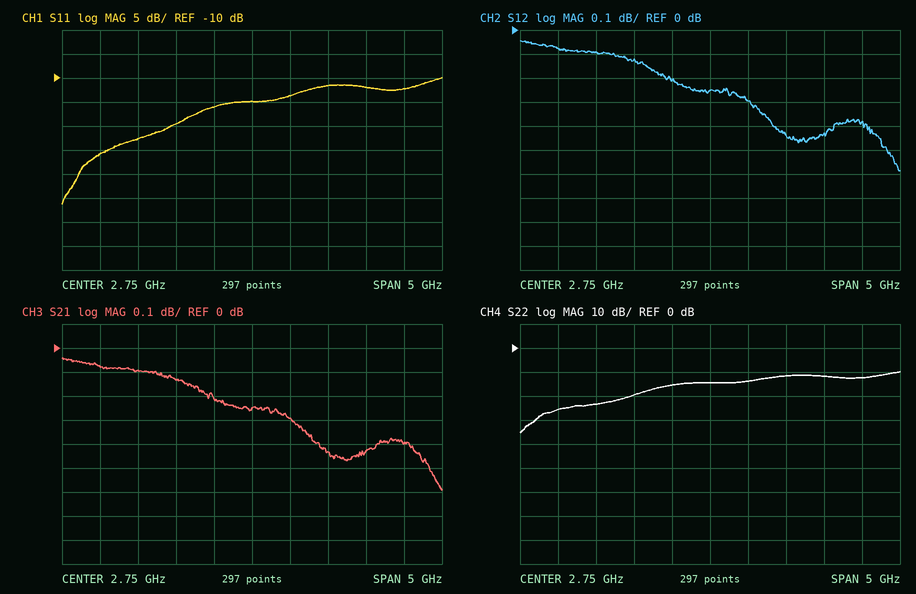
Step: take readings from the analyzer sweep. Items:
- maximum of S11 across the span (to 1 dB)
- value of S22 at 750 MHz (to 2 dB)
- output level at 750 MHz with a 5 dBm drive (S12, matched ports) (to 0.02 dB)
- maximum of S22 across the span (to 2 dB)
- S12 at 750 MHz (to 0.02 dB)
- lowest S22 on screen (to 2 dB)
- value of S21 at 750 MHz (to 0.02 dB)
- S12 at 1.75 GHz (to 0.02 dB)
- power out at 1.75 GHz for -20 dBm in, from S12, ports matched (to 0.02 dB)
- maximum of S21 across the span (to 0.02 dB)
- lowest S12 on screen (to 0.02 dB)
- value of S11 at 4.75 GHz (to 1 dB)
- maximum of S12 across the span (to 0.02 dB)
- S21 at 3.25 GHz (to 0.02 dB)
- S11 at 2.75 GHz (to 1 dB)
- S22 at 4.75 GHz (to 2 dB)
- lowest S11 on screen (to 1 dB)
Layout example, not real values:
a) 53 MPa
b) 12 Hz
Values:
a) -10 dB
b) -26 dB
c) 4.92 dBm
d) -10 dB
e) -0.08 dB
f) -36 dB
g) -0.08 dB
h) -0.12 dB
i) -20.12 dBm
j) -0.04 dB
k) -0.58 dB
l) -12 dB
m) -0.04 dB
n) -0.30 dB
o) -15 dB
p) -12 dB
q) -36 dB
